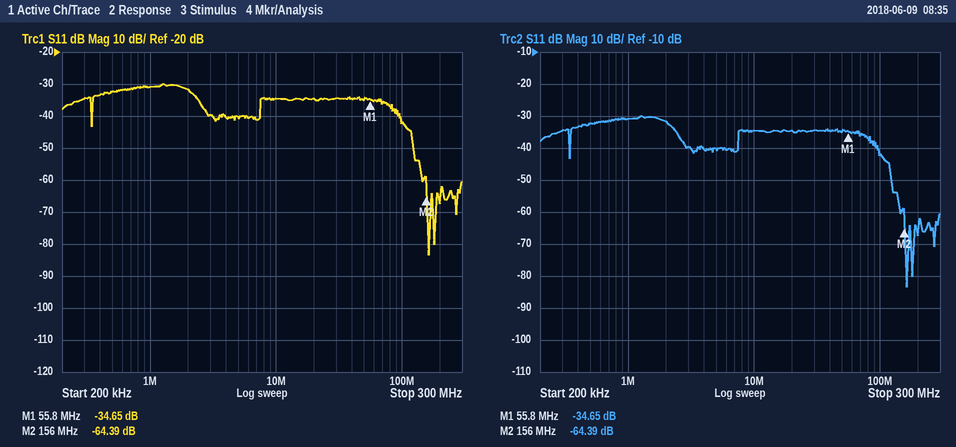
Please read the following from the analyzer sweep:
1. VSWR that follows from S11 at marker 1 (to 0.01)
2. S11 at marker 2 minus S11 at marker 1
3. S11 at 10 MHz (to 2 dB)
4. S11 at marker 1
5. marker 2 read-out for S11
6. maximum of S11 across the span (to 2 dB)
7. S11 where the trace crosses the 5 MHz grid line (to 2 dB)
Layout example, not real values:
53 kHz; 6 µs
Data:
1.04; -29.74 dB; -34 dB; -34.65 dB; -64.39 dB; -30 dB; -40 dB
